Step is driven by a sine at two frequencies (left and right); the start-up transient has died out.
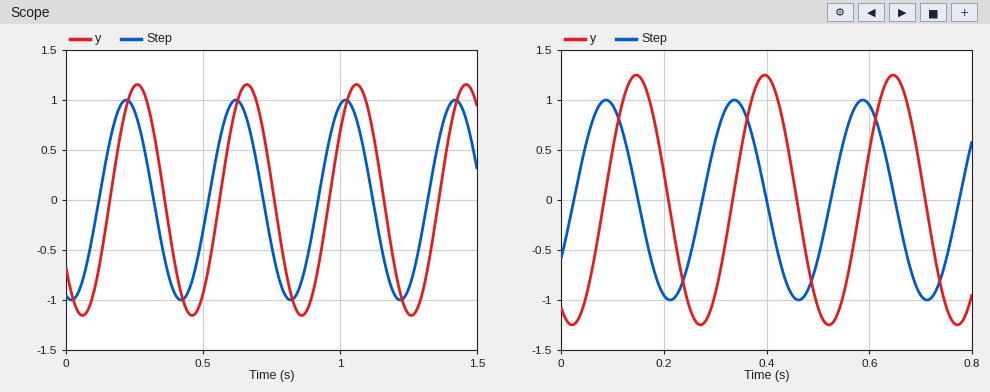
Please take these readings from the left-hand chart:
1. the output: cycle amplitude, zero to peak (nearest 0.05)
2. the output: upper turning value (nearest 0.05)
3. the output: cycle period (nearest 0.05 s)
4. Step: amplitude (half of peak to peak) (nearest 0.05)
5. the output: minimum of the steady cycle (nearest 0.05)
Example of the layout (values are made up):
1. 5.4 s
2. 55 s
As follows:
1. 1.15
2. 1.15
3. 0.40 s
4. 1.00
5. -1.15
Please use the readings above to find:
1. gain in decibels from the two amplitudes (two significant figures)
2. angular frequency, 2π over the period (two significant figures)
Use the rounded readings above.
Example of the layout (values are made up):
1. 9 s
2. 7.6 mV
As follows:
1. 1.2 dB
2. 16 rad/s
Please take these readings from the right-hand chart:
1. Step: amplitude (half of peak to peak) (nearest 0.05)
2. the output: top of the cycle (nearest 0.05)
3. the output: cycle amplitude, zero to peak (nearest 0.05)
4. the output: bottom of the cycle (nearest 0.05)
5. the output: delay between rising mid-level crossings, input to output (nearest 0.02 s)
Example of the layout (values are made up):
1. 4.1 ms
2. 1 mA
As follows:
1. 1.00
2. 1.25
3. 1.25
4. -1.25
5. 0.06 s
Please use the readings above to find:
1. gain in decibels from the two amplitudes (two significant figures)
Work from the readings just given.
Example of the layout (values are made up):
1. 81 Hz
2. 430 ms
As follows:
1. 1.9 dB
